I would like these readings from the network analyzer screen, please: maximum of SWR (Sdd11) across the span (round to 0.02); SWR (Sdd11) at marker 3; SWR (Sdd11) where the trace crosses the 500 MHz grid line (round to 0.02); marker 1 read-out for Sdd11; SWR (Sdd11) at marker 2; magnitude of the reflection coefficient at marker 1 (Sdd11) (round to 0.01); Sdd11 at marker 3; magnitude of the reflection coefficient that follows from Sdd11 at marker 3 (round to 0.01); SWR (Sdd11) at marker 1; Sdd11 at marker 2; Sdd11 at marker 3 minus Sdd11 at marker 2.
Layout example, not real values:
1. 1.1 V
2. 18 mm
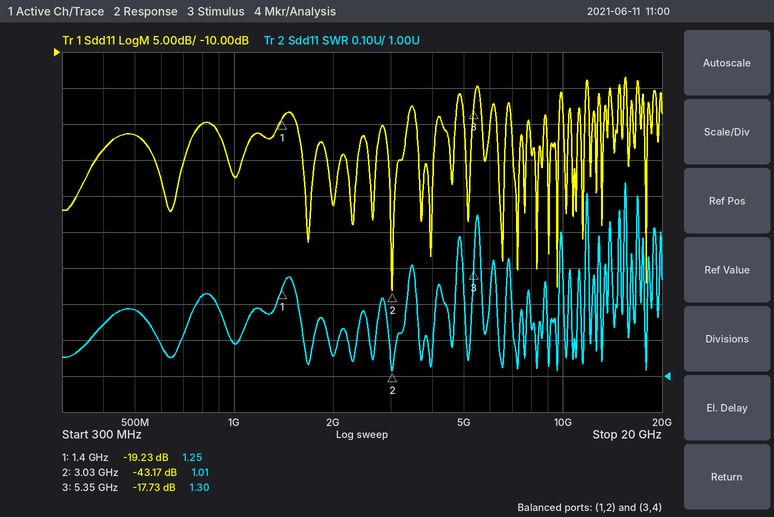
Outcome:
1. 1.54
2. 1.30
3. 1.18
4. -19.23 dB
5. 1.01
6. 0.11
7. -17.73 dB
8. 0.13
9. 1.25
10. -43.17 dB
11. 25.44 dB
